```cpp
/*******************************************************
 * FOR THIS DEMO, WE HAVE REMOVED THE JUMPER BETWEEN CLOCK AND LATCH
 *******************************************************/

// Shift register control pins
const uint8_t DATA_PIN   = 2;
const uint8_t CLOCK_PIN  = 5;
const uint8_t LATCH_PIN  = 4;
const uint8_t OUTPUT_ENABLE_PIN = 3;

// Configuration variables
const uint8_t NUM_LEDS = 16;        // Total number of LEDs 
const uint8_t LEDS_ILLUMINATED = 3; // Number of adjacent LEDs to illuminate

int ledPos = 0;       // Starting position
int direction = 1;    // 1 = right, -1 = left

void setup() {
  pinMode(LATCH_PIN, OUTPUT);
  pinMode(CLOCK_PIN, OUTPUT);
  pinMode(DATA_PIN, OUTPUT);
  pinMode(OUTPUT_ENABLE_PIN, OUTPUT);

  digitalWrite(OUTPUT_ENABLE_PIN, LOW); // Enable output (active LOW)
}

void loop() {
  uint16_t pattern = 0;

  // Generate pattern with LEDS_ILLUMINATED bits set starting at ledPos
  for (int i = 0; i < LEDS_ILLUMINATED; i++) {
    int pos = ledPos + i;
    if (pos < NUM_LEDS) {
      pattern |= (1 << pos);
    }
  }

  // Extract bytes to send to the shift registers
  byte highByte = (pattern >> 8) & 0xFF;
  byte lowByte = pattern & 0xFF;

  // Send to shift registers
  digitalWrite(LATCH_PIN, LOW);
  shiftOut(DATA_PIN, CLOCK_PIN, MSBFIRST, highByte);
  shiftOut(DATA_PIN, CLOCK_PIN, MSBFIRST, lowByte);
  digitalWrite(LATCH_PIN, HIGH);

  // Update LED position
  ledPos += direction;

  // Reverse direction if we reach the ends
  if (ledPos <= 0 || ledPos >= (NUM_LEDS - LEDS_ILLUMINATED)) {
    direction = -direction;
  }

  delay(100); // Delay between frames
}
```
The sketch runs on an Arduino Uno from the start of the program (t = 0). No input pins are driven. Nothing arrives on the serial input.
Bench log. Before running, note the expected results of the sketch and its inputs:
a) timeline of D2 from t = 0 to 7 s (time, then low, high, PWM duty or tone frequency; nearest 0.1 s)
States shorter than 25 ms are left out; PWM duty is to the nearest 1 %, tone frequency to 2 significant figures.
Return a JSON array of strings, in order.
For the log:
["0 s high; 0.1 s low; 2.6 s high; 2.7 s low; 5.2 s high; 5.3 s low"]
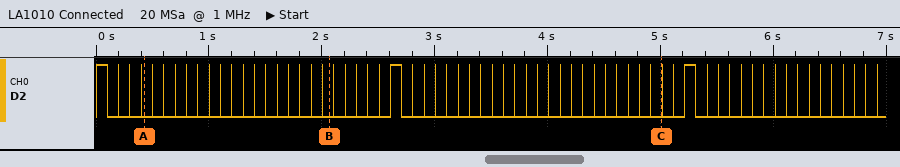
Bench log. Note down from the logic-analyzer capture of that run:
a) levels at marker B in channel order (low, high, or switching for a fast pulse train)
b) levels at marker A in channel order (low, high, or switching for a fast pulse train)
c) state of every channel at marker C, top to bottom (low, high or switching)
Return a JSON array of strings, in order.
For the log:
["D2 low", "D2 low", "D2 low"]
